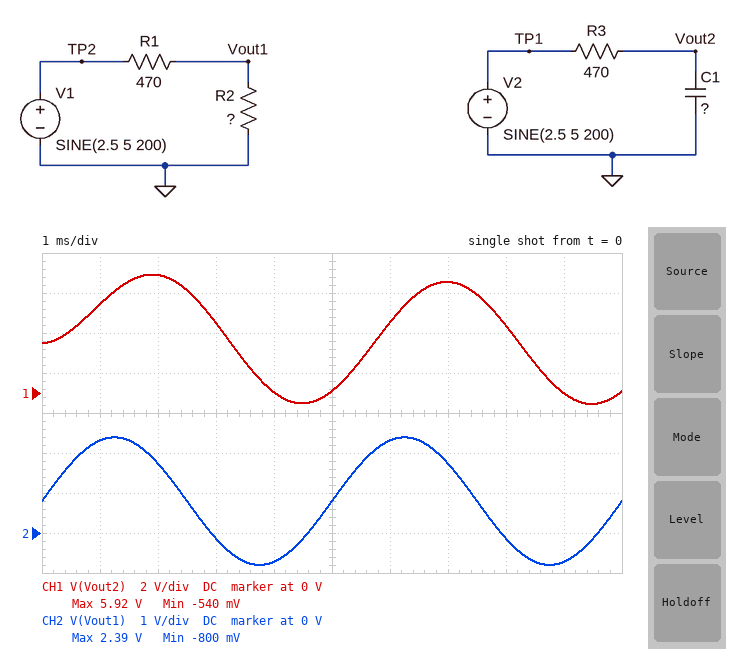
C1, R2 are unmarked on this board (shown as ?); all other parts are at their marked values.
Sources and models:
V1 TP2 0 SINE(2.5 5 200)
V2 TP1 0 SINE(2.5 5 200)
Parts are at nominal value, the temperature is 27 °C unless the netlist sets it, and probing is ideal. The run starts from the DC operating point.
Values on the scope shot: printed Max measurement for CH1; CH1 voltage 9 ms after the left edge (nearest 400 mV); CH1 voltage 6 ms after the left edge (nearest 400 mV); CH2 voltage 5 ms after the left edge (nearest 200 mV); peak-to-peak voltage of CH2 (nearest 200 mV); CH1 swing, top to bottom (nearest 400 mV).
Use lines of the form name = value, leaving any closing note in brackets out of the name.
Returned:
printed Max measurement for CH1 = 5.92 V
CH1 voltage 9 ms after the left edge = 0 V
CH1 voltage 6 ms after the left edge = 3.6 V
CH2 voltage 5 ms after the left edge = 800 mV
peak-to-peak voltage of CH2 = 3.2 V
CH1 swing, top to bottom = 6.4 V
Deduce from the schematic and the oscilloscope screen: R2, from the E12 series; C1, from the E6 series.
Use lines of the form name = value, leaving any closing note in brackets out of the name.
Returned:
R2, from the E12 series = 220 Ω
C1, from the E6 series = 2.2 µF
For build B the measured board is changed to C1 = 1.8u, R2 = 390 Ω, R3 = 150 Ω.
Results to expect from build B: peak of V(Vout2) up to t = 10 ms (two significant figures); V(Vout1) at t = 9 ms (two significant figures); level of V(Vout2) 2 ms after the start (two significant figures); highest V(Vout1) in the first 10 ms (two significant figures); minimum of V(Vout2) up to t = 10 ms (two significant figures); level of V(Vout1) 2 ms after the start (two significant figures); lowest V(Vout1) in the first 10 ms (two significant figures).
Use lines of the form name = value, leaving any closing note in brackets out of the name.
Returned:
peak of V(Vout2) up to t = 10 ms = 7.2 V
V(Vout1) at t = 9 ms = -1.0 V
level of V(Vout2) 2 ms after the start = 6.4 V
highest V(Vout1) in the first 10 ms = 3.4 V
minimum of V(Vout2) up to t = 10 ms = -2.2 V
level of V(Vout1) 2 ms after the start = 2.5 V
lowest V(Vout1) in the first 10 ms = -1.1 V
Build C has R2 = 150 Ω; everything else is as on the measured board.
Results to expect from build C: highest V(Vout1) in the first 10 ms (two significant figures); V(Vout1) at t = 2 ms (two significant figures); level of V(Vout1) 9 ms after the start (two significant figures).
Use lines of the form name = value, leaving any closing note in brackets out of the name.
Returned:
highest V(Vout1) in the first 10 ms = 1.8 V
V(Vout1) at t = 2 ms = 1.3 V
level of V(Vout1) 9 ms after the start = -550 mV
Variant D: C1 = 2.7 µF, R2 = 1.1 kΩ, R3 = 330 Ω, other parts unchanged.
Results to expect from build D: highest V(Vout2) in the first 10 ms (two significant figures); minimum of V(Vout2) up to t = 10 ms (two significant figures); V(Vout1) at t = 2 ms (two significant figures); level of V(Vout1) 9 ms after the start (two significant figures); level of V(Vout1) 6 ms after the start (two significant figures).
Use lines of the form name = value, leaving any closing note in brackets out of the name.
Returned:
highest V(Vout2) in the first 10 ms = 6.1 V
minimum of V(Vout2) up to t = 10 ms = -830 mV
V(Vout1) at t = 2 ms = 3.8 V
level of V(Vout1) 9 ms after the start = -1.6 V
level of V(Vout1) 6 ms after the start = 5.1 V
